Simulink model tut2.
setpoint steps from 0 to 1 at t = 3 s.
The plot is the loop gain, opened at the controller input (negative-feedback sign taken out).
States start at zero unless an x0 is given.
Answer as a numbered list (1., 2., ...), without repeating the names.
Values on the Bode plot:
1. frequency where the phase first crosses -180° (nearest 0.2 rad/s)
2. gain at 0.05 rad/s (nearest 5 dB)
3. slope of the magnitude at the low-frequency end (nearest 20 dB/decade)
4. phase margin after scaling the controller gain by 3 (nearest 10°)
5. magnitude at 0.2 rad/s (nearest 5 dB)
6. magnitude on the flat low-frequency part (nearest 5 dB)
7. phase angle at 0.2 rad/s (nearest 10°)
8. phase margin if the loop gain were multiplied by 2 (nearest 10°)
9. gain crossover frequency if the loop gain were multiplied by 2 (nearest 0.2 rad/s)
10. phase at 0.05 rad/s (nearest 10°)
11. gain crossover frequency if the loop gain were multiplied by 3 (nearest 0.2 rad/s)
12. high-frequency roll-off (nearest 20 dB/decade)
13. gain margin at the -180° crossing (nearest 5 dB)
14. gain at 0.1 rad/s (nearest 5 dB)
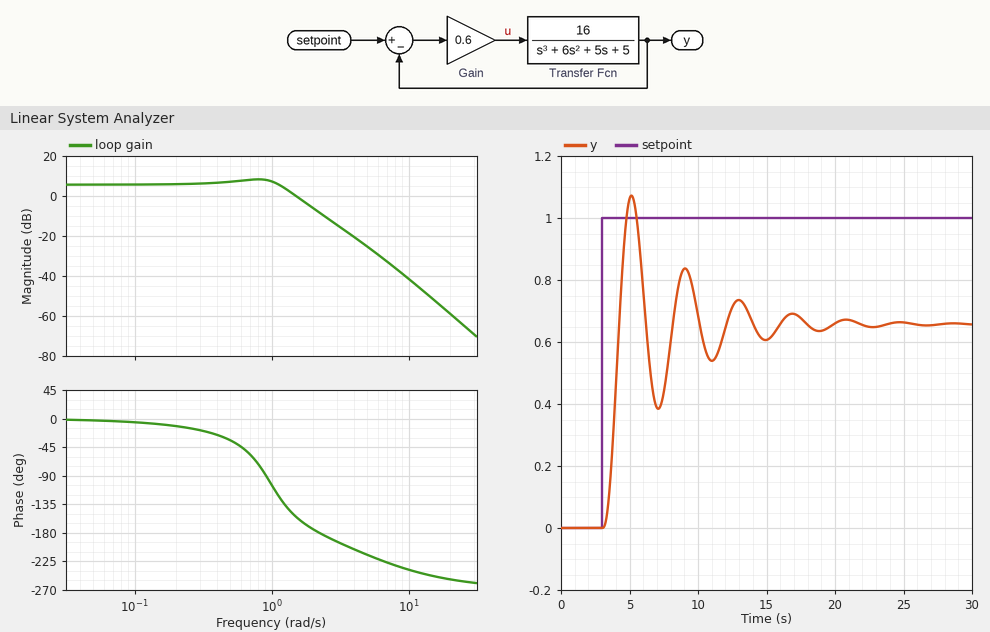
1. 2.2 rad/s
2. 5 dB
3. 0 dB/decade
4. 0°
5. 5 dB
6. 5 dB
7. -10°
8. 10°
9. 2.0 rad/s
10. 0°
11. 2.4 rad/s
12. -60 dB/decade
13. 10 dB
14. 5 dB
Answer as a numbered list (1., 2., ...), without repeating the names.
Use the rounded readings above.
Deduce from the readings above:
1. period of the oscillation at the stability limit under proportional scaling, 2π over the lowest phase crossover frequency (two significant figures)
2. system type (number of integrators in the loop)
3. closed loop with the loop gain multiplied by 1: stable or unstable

1. 2.9 s
2. 0
3. stable
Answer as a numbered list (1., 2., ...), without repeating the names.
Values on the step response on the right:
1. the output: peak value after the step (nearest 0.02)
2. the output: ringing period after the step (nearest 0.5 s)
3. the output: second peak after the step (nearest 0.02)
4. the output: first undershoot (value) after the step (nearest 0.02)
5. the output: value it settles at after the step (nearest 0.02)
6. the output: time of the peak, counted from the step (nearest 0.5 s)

1. 1.08
2. 4.0 s
3. 0.84
4. 0.38
5. 0.66
6. 2.0 s
